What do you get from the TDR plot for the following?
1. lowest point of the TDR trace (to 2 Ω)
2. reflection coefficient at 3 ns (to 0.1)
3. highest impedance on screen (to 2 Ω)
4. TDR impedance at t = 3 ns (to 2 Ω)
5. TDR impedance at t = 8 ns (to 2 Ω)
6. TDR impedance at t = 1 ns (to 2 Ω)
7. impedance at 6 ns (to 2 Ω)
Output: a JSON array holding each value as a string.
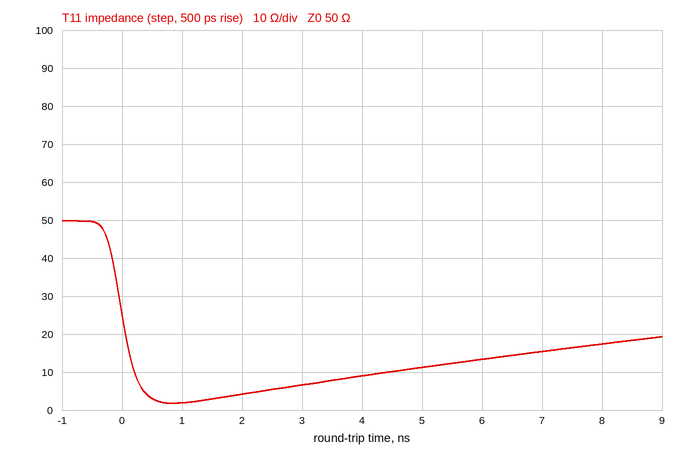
["2 Ω", "-0.8", "50 Ω", "6 Ω", "18 Ω", "2 Ω", "14 Ω"]
